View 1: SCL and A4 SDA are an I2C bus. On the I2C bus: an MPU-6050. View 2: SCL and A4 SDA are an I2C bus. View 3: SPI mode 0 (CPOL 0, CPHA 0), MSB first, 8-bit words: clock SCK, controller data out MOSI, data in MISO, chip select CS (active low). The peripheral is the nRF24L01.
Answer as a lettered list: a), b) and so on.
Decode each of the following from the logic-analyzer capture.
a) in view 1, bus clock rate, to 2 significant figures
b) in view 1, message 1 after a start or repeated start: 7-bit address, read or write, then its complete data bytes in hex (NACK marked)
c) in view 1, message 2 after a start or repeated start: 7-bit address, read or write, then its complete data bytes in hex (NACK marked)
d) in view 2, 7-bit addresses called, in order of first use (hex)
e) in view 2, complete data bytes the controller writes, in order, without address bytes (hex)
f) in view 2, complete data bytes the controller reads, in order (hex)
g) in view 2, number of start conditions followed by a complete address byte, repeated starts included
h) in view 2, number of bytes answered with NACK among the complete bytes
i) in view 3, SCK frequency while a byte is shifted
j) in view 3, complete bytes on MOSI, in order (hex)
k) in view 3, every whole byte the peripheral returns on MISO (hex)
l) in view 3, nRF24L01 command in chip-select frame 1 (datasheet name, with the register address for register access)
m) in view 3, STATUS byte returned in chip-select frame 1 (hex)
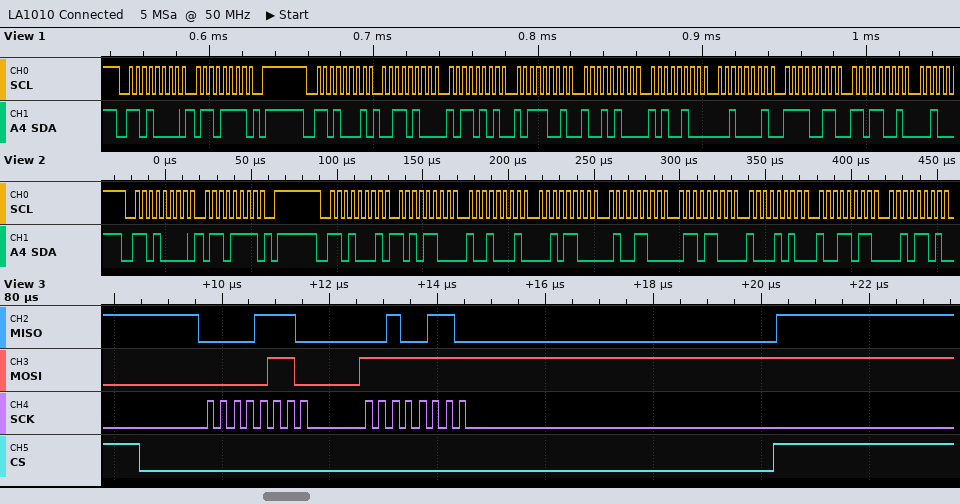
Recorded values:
a) 250 kHz
b) 0x68 write: 6F
c) 0x68 read: 34 B5 B9 94 A4 21 F3 D9
d) 0x68
e) 6F
f) AC 91 2C 4C 6C 8A 9B 2D
g) 2
h) 0
i) 4 MHz
j) 06 FF
k) 0E 26
l) R_REGISTER 0x06
m) 0x0E
